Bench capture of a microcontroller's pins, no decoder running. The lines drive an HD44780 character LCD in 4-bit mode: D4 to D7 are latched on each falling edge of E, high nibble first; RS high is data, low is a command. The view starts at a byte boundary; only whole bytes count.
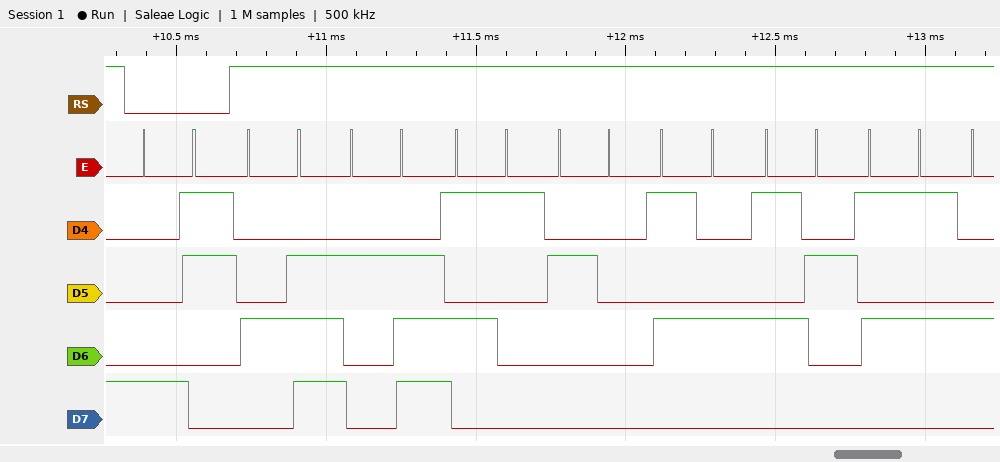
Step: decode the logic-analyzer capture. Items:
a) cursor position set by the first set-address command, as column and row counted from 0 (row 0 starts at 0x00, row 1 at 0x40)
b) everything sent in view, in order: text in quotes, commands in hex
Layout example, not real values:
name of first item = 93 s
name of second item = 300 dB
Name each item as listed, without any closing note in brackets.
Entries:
cursor position set by the first set-address command, as column and row counted from 0 = column 3, row 0
everything sent in view, in order: text in quotes, commands in hex = 0x83 "N.Q TRU"
